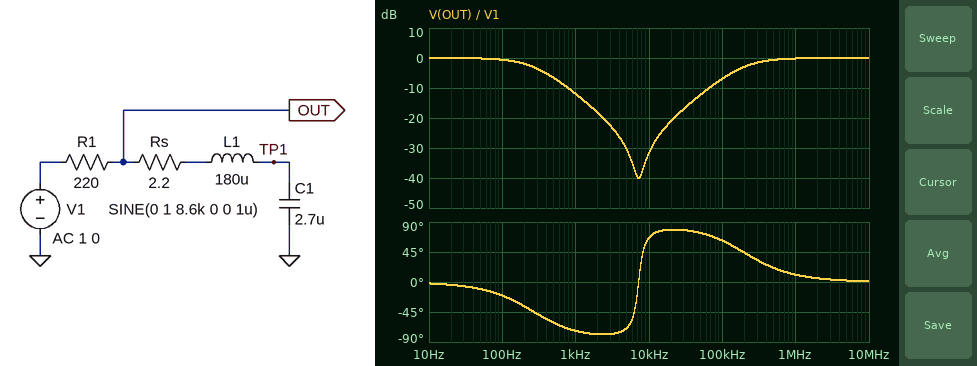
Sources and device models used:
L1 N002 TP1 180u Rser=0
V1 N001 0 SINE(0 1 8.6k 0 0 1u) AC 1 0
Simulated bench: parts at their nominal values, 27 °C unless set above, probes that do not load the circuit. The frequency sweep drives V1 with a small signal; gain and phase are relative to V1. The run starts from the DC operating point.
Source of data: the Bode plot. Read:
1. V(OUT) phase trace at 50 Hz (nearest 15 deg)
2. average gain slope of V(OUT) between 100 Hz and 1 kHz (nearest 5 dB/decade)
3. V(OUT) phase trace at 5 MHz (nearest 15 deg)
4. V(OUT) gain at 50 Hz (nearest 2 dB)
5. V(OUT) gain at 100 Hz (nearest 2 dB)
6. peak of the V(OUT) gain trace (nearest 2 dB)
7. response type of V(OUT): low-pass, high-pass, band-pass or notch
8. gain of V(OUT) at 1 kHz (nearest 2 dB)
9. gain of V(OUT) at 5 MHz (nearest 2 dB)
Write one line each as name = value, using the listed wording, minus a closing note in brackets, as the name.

V(OUT) phase trace at 50 Hz = -15 deg
average gain slope of V(OUT) between 100 Hz and 1 kHz = -10 dB/decade
V(OUT) phase trace at 5 MHz = 0 deg
V(OUT) gain at 50 Hz = 0 dB
V(OUT) gain at 100 Hz = 0 dB
peak of the V(OUT) gain trace = 0 dB
response type of V(OUT): low-pass, high-pass, band-pass or notch = notch
gain of V(OUT) at 1 kHz = -12 dB
gain of V(OUT) at 5 MHz = 0 dB
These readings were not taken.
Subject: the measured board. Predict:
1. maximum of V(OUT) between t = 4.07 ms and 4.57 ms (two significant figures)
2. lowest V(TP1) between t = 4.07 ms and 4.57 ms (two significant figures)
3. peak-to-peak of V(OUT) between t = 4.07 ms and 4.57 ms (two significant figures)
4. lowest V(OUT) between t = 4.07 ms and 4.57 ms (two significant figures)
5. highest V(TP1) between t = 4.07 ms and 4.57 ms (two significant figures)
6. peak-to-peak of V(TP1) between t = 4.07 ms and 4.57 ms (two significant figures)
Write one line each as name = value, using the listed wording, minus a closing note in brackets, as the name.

maximum of V(OUT) between t = 4.07 ms and 4.57 ms = 16 mV
lowest V(TP1) between t = 4.07 ms and 4.57 ms = -31 mV
peak-to-peak of V(OUT) between t = 4.07 ms and 4.57 ms = 33 mV
lowest V(OUT) between t = 4.07 ms and 4.57 ms = -16 mV
highest V(TP1) between t = 4.07 ms and 4.57 ms = 31 mV
peak-to-peak of V(TP1) between t = 4.07 ms and 4.57 ms = 62 mV
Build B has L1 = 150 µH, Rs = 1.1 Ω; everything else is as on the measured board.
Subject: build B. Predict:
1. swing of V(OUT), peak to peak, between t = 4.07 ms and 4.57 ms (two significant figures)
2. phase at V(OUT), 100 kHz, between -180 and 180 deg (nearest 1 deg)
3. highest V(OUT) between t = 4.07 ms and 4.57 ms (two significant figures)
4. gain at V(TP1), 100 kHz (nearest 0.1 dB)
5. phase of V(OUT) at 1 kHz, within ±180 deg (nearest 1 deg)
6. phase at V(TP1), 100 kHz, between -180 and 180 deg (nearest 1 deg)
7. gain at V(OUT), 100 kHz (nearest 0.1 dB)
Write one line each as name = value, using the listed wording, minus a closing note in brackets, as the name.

swing of V(OUT), peak to peak, between t = 4.07 ms and 4.57 ms = 15 mV
phase at V(OUT), 100 kHz, between -180 and 180 deg = 66 deg
highest V(OUT) between t = 4.07 ms and 4.57 ms = 7.6 mV
gain at V(TP1), 100 kHz = -52.2 dB
phase of V(OUT) at 1 kHz, within ±180 deg = -74 deg
phase at V(TP1), 100 kHz, between -180 and 180 deg = -113 deg
gain at V(OUT), 100 kHz = -8.2 dB
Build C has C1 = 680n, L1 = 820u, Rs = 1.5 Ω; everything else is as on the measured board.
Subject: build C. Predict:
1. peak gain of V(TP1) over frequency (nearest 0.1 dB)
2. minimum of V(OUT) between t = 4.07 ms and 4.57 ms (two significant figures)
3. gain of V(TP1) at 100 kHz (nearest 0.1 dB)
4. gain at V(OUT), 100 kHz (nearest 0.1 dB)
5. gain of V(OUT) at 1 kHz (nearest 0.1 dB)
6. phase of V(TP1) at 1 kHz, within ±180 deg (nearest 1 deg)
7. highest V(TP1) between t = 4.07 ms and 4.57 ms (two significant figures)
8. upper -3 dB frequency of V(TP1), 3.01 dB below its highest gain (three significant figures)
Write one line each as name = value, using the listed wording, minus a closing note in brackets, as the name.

peak gain of V(TP1) over frequency = 0 dB
minimum of V(OUT) between t = 4.07 ms and 4.57 ms = -77 mV
gain of V(TP1) at 100 kHz = -47.6 dB
gain at V(OUT), 100 kHz = -0.7 dB
gain of V(OUT) at 1 kHz = -2.9 dB
phase of V(TP1) at 1 kHz, within ±180 deg = -44 deg
highest V(TP1) between t = 4.07 ms and 4.57 ms = 120 mV
upper -3 dB frequency of V(TP1), 3.01 dB below its highest gain = 1.08 kHz
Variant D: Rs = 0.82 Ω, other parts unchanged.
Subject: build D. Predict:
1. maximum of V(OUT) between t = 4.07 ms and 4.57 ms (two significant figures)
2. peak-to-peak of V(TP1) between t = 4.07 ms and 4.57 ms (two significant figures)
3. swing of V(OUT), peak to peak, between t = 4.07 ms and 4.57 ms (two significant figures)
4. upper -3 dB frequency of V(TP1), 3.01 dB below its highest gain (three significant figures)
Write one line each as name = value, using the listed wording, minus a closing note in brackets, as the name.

maximum of V(OUT) between t = 4.07 ms and 4.57 ms = 14 mV
peak-to-peak of V(TP1) between t = 4.07 ms and 4.57 ms = 62 mV
swing of V(OUT), peak to peak, between t = 4.07 ms and 4.57 ms = 27 mV
upper -3 dB frequency of V(TP1), 3.01 dB below its highest gain = 267 Hz
